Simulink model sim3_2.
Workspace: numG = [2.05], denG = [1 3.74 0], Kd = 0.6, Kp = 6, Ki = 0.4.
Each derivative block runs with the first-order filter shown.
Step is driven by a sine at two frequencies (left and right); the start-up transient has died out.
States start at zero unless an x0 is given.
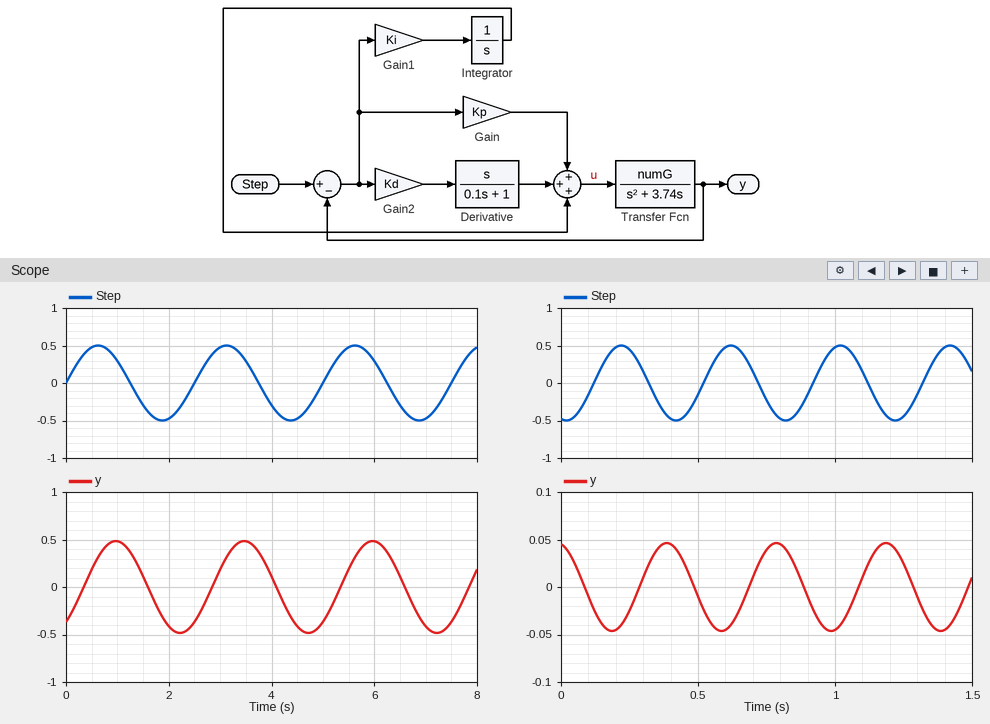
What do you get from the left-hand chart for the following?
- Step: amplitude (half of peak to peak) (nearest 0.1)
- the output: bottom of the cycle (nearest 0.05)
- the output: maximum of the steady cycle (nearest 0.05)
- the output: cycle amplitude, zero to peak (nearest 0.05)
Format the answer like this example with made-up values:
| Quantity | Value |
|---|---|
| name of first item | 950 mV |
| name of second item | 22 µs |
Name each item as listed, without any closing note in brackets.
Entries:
| Quantity | Value |
|---|---|
| Step: amplitude (half of peak to peak) | 0.5 |
| the output: bottom of the cycle | -0.50 |
| the output: maximum of the steady cycle | 0.50 |
| the output: cycle amplitude, zero to peak | 0.50 |
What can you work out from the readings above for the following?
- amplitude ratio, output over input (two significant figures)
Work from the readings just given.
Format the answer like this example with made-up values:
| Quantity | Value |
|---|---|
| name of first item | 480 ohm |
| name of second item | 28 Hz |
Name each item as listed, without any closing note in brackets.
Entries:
| Quantity | Value |
|---|---|
| amplitude ratio, output over input | 1.0 |
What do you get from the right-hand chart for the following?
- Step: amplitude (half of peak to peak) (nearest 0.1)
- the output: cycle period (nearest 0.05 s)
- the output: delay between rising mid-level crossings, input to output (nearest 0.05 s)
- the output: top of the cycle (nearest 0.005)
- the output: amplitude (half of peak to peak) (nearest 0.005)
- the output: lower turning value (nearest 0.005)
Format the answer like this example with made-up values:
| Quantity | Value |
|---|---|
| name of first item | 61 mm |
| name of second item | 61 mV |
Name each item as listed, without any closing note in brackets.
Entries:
| Quantity | Value |
|---|---|
| Step: amplitude (half of peak to peak) | 0.5 |
| the output: cycle period | 0.40 s |
| the output: delay between rising mid-level crossings, input to output | 0.15 s |
| the output: top of the cycle | 0.045 |
| the output: amplitude (half of peak to peak) | 0.045 |
| the output: lower turning value | -0.045 |
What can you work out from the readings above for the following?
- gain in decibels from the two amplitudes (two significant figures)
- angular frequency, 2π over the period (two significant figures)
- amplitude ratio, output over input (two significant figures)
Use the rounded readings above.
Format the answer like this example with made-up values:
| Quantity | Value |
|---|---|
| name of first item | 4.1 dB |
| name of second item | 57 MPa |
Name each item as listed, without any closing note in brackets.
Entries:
| Quantity | Value |
|---|---|
| gain in decibels from the two amplitudes | -21 dB |
| angular frequency, 2π over the period | 16 rad/s |
| amplitude ratio, output over input | 0.090 |
